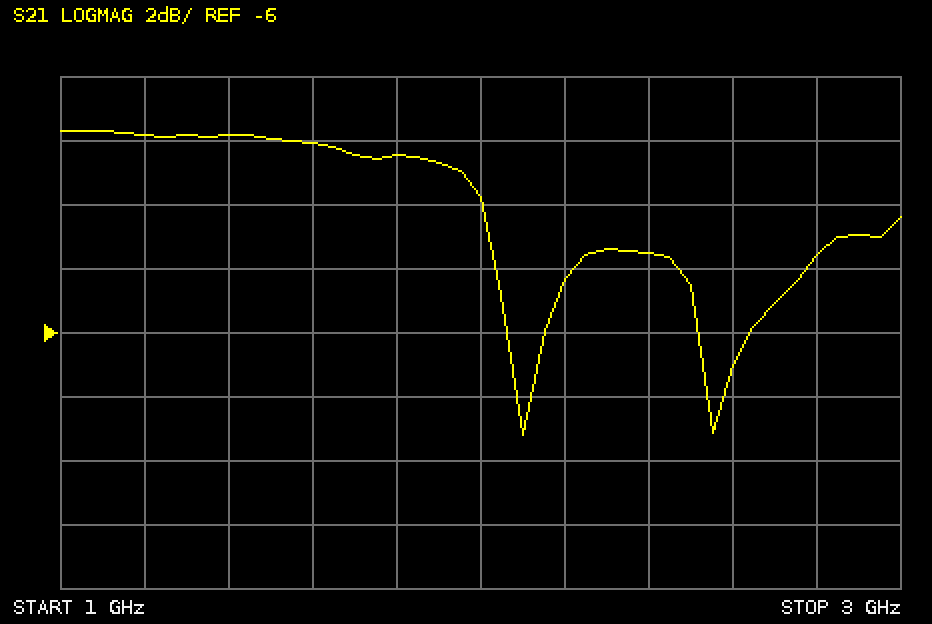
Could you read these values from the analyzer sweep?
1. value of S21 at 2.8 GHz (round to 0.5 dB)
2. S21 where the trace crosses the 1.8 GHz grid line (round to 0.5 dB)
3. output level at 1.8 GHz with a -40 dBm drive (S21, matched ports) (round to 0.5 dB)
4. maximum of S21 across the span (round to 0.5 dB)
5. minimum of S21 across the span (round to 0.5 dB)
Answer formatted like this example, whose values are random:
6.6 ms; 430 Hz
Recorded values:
-3.5 dB; -0.5 dB; -40.5 dBm; 0.5 dB; -9.0 dB
